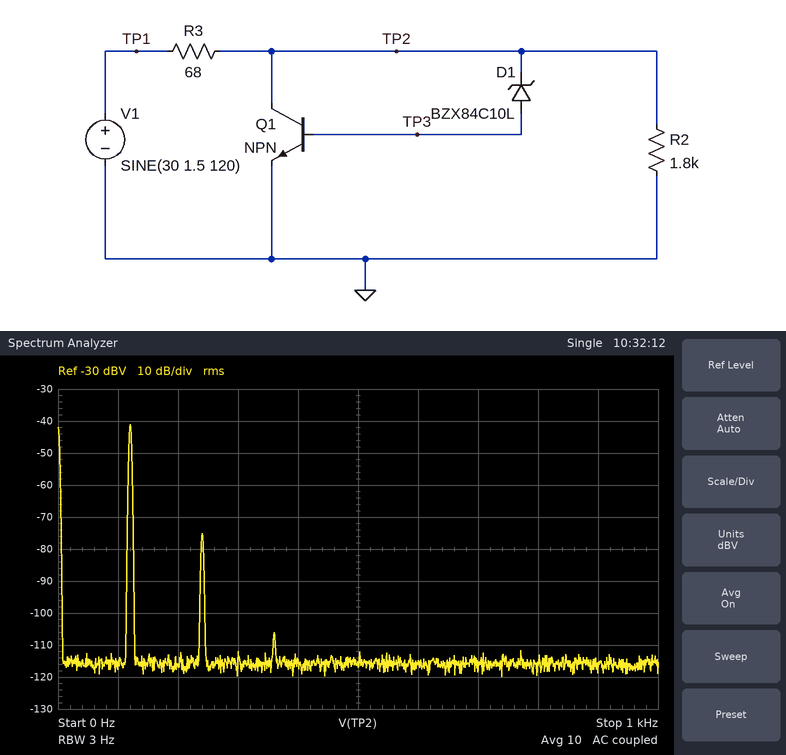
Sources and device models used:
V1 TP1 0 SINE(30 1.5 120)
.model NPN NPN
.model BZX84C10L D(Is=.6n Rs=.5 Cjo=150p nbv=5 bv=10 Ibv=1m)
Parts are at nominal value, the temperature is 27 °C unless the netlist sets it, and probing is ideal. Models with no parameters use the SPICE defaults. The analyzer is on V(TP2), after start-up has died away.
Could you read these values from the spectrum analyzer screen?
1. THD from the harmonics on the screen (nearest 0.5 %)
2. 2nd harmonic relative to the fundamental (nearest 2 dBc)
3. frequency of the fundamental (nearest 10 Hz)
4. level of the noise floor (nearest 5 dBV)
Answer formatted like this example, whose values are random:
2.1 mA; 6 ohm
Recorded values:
2.0 %; -34 dBc; 120 Hz; -115 dBV
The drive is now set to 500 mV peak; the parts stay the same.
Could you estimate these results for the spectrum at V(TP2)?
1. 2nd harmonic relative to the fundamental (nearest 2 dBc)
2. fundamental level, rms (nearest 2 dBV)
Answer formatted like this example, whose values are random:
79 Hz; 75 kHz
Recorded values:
-44 dBc; -50 dBV
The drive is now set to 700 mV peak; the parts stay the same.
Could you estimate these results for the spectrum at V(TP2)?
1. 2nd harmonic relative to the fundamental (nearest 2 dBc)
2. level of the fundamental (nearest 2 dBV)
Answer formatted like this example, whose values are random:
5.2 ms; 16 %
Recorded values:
-40 dBc; -48 dBV
